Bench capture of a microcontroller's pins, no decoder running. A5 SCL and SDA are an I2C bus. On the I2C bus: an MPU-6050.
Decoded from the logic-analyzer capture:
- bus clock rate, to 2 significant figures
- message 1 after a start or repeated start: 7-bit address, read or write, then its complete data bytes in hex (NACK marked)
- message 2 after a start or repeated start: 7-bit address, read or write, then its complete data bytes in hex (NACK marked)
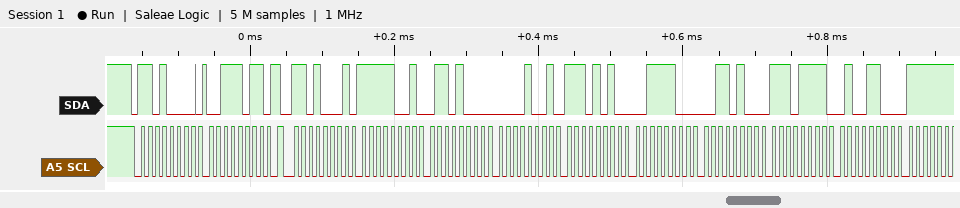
100 kHz
0x68 write: 3B
0x68 read: F9 68 09 EA 3C 34 EF 4C
